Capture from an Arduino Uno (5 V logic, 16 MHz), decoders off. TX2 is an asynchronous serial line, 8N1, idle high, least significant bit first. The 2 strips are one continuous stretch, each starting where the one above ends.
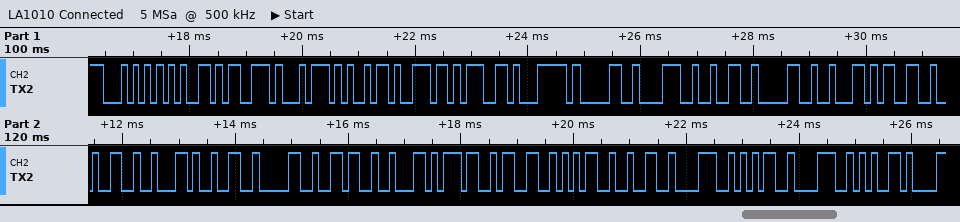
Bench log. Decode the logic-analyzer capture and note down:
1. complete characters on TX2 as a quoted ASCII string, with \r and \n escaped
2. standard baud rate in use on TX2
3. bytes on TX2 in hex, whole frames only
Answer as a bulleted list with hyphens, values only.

- "Testing|0820b32b206b7352858e"
- 9600 baud
- 54 65 73 74 69 6E 67 7C 30 38 32 30 62 33 32 62 32 30 36 62 37 33 35 32 38 35 38 65
